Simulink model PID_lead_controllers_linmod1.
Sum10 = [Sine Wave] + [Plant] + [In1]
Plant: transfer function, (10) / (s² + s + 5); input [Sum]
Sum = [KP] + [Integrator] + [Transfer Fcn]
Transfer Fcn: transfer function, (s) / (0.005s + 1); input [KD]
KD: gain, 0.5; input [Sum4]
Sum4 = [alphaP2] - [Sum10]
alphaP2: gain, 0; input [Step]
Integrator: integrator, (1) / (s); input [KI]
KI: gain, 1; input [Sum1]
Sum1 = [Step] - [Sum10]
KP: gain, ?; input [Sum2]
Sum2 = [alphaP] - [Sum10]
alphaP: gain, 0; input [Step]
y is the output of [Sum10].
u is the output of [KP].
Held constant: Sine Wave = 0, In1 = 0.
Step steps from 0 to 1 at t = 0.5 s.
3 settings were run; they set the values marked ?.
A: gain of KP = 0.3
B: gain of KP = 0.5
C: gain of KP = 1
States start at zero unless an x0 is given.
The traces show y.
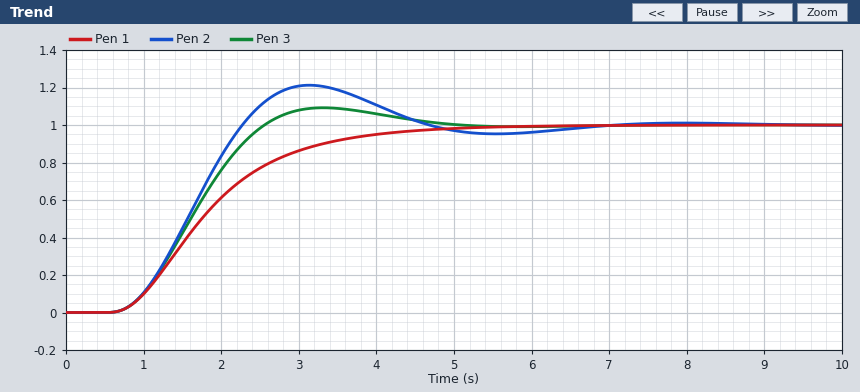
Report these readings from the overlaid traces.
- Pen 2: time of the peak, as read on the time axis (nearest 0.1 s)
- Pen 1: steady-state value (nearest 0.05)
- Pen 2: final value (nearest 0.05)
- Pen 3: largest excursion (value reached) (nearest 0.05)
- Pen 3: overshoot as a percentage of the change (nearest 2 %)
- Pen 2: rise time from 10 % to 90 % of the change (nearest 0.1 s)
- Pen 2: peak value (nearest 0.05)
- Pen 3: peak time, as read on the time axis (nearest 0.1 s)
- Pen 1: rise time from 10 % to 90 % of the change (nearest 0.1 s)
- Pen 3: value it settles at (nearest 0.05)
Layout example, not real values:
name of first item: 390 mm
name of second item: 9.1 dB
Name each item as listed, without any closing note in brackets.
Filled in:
Pen 2: time of the peak, as read on the time axis: 3.1 s
Pen 1: steady-state value: 1.00
Pen 2: final value: 1.00
Pen 3: largest excursion (value reached): 1.10
Pen 3: overshoot as a percentage of the change: 10 %
Pen 2: rise time from 10 % to 90 % of the change: 1.1 s
Pen 2: peak value: 1.20
Pen 3: peak time, as read on the time axis: 3.3 s
Pen 1: rise time from 10 % to 90 % of the change: 2.3 s
Pen 3: value it settles at: 1.00
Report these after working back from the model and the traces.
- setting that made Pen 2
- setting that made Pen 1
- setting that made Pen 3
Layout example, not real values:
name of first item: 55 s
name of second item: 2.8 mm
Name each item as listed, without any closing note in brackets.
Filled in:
setting that made Pen 2: A
setting that made Pen 1: C
setting that made Pen 3: B
